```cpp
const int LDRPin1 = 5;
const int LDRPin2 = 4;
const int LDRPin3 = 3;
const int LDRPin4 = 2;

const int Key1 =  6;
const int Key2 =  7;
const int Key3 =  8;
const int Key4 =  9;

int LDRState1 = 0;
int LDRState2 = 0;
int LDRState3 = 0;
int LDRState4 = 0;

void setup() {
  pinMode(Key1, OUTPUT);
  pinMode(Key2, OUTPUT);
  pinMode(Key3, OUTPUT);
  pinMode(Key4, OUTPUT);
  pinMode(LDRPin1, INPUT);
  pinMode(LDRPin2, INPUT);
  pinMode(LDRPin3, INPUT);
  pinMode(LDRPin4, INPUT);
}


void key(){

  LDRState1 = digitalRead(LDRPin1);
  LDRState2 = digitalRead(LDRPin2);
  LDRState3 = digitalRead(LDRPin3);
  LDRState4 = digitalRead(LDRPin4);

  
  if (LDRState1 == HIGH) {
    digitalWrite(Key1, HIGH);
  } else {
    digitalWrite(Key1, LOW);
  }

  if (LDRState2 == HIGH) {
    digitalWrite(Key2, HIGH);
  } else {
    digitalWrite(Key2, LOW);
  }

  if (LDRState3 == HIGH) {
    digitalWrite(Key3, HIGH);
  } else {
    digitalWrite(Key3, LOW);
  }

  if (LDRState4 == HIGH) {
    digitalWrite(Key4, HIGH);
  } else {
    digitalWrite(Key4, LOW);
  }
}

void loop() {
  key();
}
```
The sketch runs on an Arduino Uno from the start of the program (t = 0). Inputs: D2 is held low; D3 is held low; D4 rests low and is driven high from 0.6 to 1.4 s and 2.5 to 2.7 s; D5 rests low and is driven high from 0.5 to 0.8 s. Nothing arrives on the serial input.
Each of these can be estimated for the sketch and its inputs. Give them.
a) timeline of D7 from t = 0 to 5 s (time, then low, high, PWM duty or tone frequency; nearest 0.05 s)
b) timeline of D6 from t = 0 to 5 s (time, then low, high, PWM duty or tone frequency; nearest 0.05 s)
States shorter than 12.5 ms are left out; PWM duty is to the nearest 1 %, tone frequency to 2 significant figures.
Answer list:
0 s low; 0.6 s high; 1.4 s low; 2.5 s high; 2.7 s low
0 s low; 0.5 s high; 0.8 s low
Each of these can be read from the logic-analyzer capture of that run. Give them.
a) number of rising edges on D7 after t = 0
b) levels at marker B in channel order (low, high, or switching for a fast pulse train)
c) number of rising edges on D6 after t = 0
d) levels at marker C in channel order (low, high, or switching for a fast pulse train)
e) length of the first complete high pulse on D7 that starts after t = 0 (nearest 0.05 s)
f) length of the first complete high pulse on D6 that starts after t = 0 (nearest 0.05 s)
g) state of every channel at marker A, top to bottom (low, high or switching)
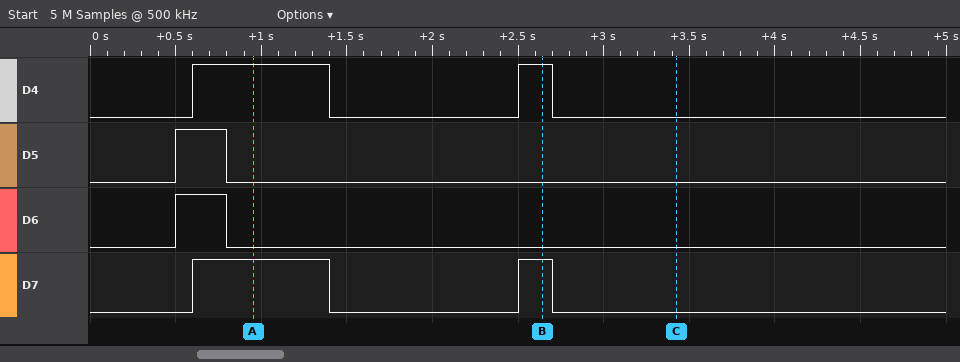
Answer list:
2
D4 high, D5 low, D6 low, D7 high
1
D4 low, D5 low, D6 low, D7 low
0.80 s
0.30 s
D4 high, D5 low, D6 low, D7 high
